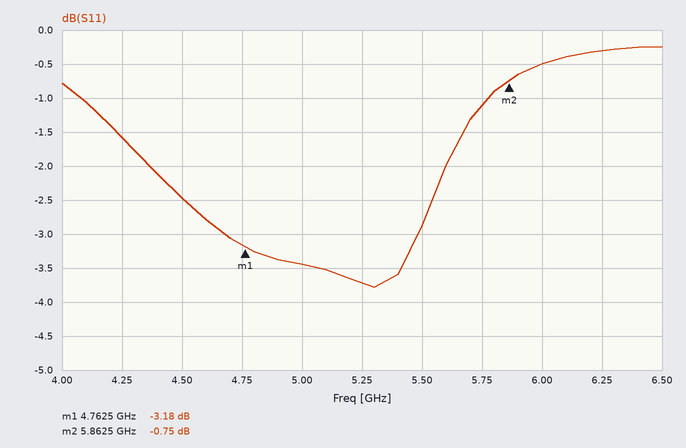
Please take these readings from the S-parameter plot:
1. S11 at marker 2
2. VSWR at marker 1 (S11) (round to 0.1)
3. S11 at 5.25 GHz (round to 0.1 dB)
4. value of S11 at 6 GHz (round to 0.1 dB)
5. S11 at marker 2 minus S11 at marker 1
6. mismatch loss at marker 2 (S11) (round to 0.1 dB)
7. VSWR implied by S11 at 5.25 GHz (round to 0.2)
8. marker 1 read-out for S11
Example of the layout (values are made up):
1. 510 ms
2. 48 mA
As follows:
1. -0.75 dB
2. 5.5
3. -3.7 dB
4. -0.5 dB
5. 2.43 dB
6. 8.0 dB
7. 4.8
8. -3.18 dB
